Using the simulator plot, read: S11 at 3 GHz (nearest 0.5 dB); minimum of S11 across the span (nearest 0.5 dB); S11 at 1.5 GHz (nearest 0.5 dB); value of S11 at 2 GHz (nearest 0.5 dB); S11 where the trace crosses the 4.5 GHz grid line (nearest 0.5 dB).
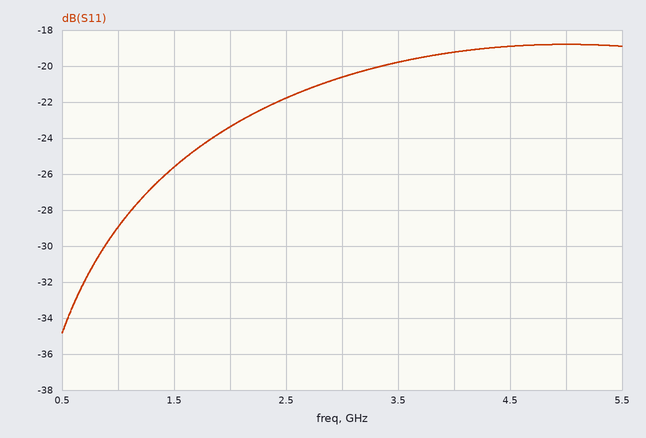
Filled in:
-20.5 dB
-35.0 dB
-25.5 dB
-23.5 dB
-19.0 dB
